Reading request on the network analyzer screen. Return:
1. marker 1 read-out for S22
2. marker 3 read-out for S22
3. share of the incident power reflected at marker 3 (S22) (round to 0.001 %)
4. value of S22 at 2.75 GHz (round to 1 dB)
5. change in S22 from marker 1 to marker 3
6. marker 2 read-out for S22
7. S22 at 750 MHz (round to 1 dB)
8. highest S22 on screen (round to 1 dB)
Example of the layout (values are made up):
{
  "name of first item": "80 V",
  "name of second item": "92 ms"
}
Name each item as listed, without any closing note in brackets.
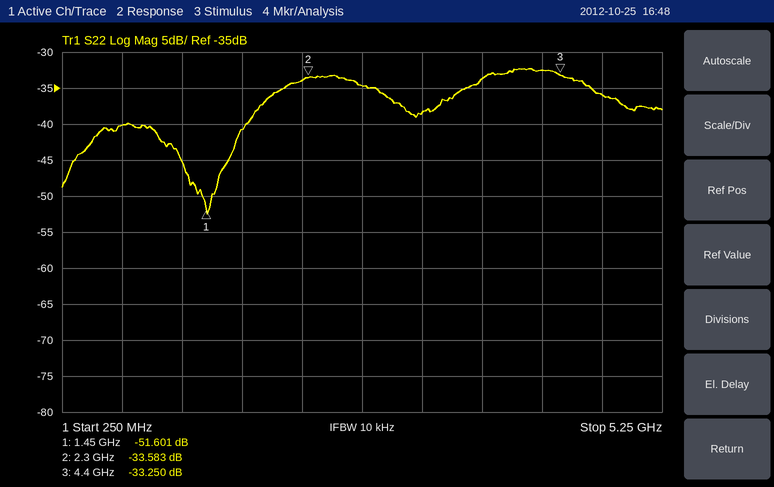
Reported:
{
  "marker 1 read-out for S22": "-51.601 dB",
  "marker 3 read-out for S22": "-33.250 dB",
  "share of the incident power reflected at marker 3 (S22)": "0.047 %",
  "value of S22 at 2.75 GHz": "-35 dB",
  "change in S22 from marker 1 to marker 3": "18.351 dB",
  "marker 2 read-out for S22": "-33.583 dB",
  "S22 at 750 MHz": "-40 dB",
  "highest S22 on screen": "-32 dB"
}
